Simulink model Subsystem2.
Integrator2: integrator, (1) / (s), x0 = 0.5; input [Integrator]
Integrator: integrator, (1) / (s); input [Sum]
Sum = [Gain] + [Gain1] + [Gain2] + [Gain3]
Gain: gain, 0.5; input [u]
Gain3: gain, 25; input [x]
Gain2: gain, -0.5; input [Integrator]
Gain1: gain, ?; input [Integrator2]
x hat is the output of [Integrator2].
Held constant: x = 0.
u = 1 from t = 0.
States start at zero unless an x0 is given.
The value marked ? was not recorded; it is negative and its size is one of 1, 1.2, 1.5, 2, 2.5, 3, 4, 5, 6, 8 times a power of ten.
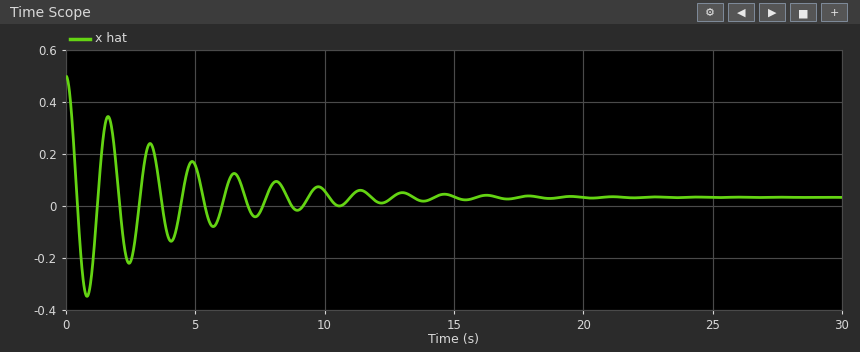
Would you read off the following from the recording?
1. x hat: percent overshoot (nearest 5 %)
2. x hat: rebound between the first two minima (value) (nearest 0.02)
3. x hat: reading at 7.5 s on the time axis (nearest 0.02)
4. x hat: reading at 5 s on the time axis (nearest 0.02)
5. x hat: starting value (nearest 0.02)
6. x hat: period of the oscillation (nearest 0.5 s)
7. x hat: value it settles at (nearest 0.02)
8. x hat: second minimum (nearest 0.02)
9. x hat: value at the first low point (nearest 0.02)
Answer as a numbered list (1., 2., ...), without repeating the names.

1. 80 %
2. 0.34
3. -0.02
4. 0.16
5. 0.50
6. 1.5 s
7. 0.04
8. -0.22
9. -0.34
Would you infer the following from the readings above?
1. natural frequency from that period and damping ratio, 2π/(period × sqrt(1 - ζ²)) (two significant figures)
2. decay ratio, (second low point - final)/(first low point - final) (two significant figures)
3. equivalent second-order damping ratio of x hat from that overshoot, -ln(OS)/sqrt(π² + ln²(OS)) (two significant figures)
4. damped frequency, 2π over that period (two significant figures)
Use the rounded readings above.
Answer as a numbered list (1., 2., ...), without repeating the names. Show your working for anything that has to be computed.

1. 2π / (1.5 × sqrt(1 - 0.071²)) = 4.2 rad/s
2. (-0.22 - 0.04) / (-0.34 - 0.04) = 0.68
3. ln(0.8) = -0.223; 0.223 / sqrt(9.870 + 0.050) = 0.071
4. 2π / 1.5 = 4.2 rad/s
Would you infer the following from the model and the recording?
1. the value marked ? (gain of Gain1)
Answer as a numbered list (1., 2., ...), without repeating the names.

1. -15
